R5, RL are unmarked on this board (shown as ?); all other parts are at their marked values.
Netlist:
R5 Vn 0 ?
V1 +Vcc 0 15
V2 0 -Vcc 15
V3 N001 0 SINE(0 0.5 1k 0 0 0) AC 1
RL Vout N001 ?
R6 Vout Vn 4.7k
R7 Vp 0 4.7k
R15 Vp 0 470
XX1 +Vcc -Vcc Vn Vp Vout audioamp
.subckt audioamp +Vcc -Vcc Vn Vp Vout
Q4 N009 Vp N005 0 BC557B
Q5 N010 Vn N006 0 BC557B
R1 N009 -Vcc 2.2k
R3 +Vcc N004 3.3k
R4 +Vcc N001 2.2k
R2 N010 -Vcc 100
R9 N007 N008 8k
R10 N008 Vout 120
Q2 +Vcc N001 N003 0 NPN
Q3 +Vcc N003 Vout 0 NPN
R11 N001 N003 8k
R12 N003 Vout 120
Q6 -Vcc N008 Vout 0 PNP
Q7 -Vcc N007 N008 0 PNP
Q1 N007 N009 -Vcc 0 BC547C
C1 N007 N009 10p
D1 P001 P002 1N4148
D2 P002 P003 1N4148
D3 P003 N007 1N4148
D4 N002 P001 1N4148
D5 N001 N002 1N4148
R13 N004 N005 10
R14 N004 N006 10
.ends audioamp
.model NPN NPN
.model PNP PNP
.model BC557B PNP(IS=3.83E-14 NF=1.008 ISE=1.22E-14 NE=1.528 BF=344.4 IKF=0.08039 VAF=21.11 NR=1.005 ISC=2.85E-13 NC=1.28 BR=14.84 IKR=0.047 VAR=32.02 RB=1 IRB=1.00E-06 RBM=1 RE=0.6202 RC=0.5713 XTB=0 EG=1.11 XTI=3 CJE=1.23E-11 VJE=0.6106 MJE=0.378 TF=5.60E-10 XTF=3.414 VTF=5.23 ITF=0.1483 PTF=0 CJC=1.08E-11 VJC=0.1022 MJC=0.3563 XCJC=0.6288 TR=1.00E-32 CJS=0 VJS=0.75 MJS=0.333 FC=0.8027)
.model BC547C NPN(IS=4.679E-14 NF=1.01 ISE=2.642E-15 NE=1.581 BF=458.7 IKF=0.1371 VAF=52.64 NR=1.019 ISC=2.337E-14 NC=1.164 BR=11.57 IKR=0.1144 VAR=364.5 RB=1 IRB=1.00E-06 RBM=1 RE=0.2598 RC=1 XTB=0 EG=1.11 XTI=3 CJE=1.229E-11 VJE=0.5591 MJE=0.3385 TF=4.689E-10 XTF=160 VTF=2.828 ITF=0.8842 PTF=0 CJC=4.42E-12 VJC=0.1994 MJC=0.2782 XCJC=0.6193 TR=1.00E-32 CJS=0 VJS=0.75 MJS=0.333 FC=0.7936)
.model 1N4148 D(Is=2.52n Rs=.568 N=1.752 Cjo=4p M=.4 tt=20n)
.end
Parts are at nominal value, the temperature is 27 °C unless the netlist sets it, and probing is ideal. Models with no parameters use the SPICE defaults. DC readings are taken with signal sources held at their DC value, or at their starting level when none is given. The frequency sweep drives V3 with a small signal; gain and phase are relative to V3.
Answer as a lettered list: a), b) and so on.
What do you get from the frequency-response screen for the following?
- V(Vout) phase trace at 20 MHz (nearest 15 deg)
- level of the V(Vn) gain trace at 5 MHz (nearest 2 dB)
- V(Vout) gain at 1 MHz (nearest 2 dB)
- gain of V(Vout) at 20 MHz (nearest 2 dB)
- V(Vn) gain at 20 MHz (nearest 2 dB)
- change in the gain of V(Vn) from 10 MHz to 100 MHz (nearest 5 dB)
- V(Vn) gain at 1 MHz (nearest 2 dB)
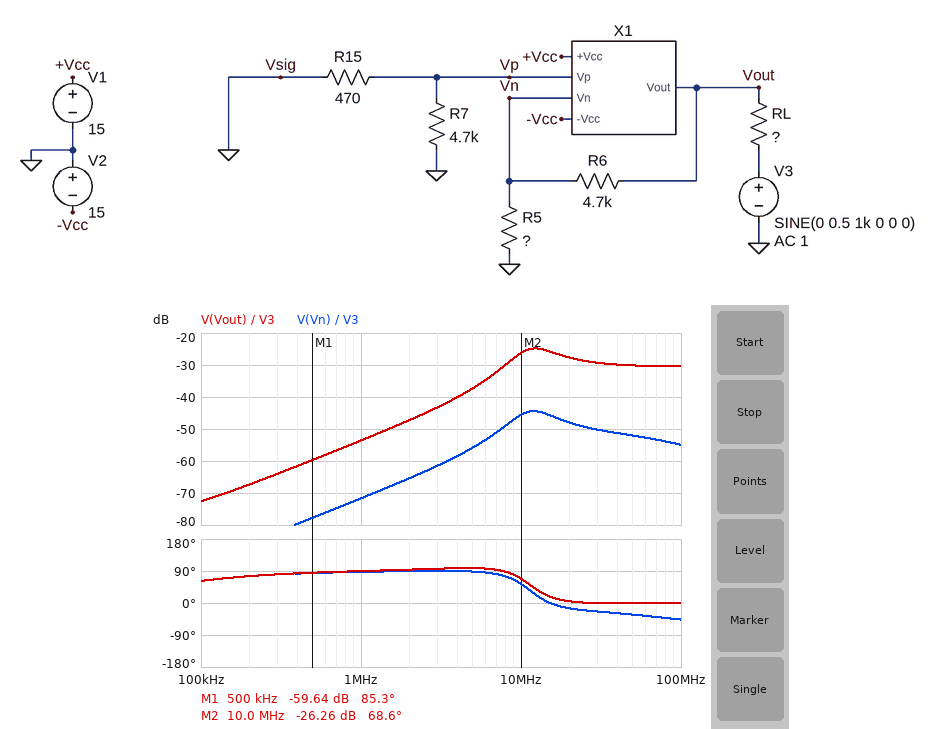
a) 0 deg
b) -56 dB
c) -54 dB
d) -28 dB
e) -48 dB
f) -10 dB
g) -72 dB
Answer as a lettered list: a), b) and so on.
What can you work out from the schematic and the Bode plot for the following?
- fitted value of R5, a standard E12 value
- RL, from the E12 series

a) 680 Ω
b) 10 Ω
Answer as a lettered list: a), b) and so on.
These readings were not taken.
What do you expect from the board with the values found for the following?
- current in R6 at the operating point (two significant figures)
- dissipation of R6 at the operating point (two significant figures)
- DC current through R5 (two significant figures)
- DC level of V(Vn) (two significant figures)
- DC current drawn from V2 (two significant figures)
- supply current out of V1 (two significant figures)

a) 160 µA
b) 130 µW
c) 160 µA
d) -110 mV
e) 110 mA
f) 22 mA
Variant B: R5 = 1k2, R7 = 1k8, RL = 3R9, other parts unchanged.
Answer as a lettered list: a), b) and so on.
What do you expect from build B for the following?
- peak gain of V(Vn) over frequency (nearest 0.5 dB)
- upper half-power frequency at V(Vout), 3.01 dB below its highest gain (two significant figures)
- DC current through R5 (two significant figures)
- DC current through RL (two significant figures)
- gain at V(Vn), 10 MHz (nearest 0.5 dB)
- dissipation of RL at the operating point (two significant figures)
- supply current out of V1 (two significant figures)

a) -33.5 dB
b) 18 MHz
c) 89 µA
d) 140 mA
e) -39.5 dB
f) 80 mW
g) 19 mA
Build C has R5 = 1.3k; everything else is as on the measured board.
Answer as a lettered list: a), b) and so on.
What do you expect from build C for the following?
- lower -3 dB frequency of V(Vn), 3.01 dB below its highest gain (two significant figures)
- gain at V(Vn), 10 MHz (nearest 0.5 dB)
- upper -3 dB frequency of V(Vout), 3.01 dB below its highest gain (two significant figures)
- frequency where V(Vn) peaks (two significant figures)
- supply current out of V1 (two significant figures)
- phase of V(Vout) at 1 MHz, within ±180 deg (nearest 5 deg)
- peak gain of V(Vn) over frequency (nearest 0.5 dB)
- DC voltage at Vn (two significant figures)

a) 11 MHz
b) -40.5 dB
c) 17 MHz
d) 13 MHz
e) 23 mA
f) 95 deg
g) -34.0 dB
h) -110 mV
